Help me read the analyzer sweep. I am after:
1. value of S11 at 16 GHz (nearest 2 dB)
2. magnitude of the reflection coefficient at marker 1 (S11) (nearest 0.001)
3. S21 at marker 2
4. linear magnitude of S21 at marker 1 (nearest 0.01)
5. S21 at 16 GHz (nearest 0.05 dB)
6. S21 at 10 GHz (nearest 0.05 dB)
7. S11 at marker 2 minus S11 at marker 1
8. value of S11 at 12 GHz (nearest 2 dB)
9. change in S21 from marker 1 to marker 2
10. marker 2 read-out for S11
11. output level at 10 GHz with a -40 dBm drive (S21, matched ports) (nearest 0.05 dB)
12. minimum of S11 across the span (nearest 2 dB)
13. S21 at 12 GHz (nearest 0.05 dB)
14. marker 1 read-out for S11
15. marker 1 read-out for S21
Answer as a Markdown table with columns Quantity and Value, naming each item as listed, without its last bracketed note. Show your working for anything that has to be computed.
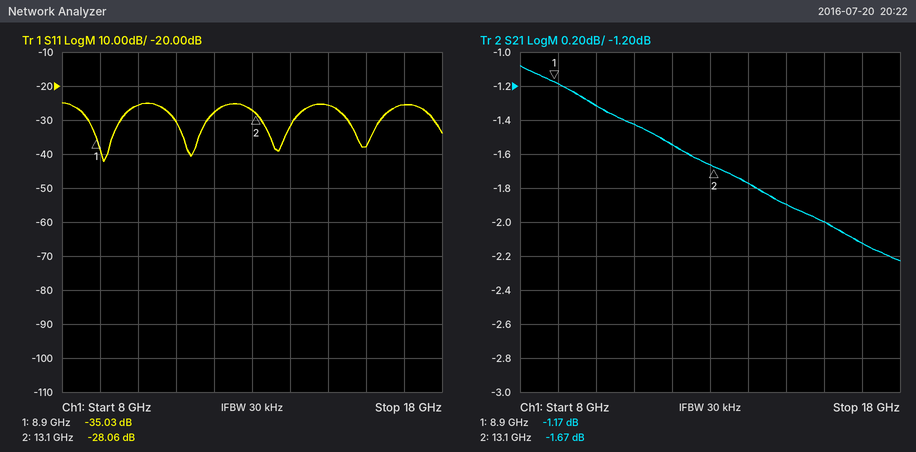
| Quantity | Value |
|---|---|
| value of S11 at 16 GHz | -38 dB |
| magnitude of the reflection coefficient at marker 1 (S11) | 10^(-35.03/20) ≈ 0.018 |
| S21 at marker 2 | -1.67 dB |
| linear magnitude of S21 at marker 1 | 10^(-1.17/20) ≈ 0.87 |
| S21 at 16 GHz | -2.00 dB |
| S21 at 10 GHz | -1.30 dB |
| S11 at marker 2 minus S11 at marker 1 | -28.06 − (-35.03) = 6.97 dB |
| value of S11 at 12 GHz | -28 dB |
| change in S21 from marker 1 to marker 2 | -1.67 − (-1.17) = -0.50 dB |
| marker 2 read-out for S11 | -28.06 dB |
| output level at 10 GHz with a -40 dBm drive (S21, matched ports) | -40 dBm + (-1.30 dB) = -41.30 dBm |
| minimum of S11 across the span | -42 dB |
| S21 at 12 GHz | -1.55 dB |
| marker 1 read-out for S11 | -35.03 dB |
| marker 1 read-out for S21 | -1.17 dB |
